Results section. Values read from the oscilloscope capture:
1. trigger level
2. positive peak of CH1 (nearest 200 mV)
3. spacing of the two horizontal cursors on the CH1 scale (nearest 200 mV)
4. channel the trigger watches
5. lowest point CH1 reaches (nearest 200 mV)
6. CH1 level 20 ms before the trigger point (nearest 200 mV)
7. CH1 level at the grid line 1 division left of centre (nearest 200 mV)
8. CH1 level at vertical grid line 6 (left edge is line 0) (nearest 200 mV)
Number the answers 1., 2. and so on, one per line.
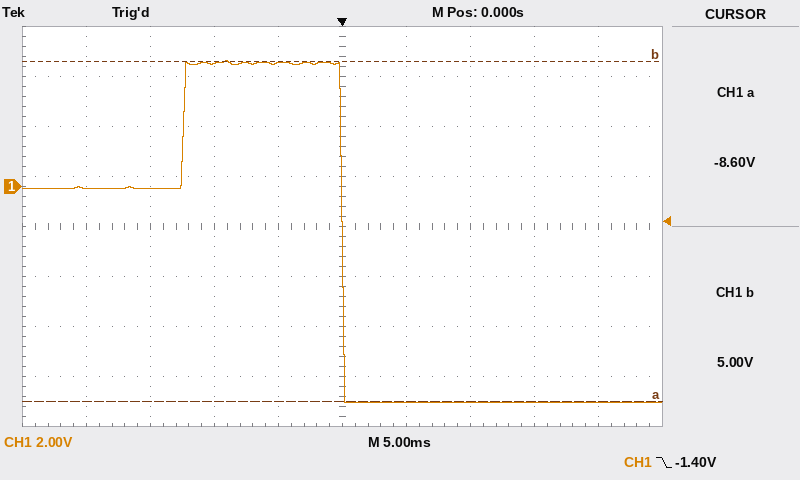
1. -1.40 V
2. 5.0 V
3. 13.6 V
4. CH1
5. -8.6 V
6. 0.0 V
7. 5.0 V
8. -8.6 V
